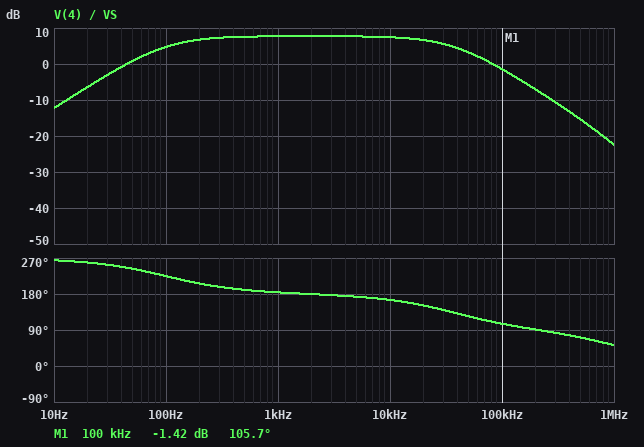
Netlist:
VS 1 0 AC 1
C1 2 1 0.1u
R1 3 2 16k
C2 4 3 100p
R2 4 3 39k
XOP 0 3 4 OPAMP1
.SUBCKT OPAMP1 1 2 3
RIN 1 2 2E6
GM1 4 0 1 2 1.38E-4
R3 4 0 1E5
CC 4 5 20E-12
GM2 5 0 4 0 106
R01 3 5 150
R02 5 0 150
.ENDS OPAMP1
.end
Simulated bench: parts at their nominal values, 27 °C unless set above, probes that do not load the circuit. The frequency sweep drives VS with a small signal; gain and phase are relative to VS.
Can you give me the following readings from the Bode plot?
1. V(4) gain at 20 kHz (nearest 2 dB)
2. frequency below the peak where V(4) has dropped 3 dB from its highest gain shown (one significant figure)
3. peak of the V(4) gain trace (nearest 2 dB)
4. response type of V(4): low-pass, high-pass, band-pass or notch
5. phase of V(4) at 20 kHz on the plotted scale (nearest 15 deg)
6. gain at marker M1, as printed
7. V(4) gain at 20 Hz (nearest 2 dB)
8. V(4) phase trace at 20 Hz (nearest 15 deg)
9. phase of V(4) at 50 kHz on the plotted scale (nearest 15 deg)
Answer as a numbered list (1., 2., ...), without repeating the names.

1. 6 dB
2. 100 Hz
3. 8 dB
4. band-pass
5. 150 deg
6. -1.42 dB
7. -6 dB
8. 255 deg
9. 120 deg
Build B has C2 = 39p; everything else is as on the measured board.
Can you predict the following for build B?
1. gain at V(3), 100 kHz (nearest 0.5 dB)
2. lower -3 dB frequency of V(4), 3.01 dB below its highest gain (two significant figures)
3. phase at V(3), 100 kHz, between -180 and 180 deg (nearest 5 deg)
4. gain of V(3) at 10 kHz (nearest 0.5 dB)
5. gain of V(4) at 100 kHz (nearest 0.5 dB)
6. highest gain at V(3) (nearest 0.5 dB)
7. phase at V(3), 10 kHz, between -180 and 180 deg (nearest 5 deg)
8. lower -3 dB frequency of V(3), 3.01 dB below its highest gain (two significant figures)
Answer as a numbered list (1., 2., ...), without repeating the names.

1. -17.0 dB
2. 99 Hz
3. 35 deg
4. -33.0 dB
5. 4.0 dB
6. -15.0 dB
7. 85 deg
8. 75 kHz
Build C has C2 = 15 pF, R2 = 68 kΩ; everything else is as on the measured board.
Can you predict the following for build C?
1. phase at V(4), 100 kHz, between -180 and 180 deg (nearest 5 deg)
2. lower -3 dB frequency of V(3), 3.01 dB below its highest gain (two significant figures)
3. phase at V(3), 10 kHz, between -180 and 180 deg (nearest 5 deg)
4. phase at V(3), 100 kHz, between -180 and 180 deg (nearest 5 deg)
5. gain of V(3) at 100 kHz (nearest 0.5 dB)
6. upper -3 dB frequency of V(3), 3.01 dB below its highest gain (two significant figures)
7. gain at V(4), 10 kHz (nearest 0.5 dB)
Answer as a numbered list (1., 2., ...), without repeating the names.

1. 130 deg
2. 85 kHz
3. 85 deg
4. 40 deg
5. -11.5 dB
6. 2.0 MHz
7. 12.5 dB
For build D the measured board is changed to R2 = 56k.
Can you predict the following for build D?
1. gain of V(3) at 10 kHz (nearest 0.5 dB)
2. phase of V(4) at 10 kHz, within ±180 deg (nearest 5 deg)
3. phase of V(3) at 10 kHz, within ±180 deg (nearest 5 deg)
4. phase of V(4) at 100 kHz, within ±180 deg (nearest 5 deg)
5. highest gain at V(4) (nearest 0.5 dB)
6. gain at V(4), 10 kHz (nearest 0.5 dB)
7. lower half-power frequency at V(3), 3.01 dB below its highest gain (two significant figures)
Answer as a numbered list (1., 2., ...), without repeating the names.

1. -30.5 dB
2. 160 deg
3. 70 deg
4. 100 deg
5. 11.0 dB
6. 10.5 dB
7. 25 kHz
